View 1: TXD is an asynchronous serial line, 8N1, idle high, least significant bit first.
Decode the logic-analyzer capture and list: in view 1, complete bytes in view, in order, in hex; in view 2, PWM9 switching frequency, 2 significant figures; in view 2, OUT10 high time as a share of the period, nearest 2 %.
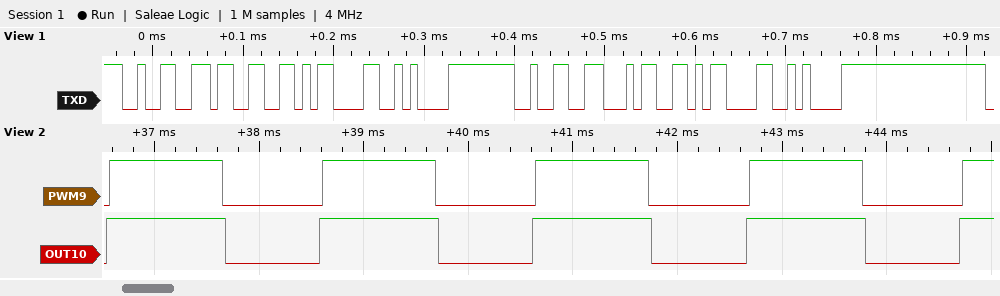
32 33 0D 0A 32 34 0D 0A
490 Hz
56 %
